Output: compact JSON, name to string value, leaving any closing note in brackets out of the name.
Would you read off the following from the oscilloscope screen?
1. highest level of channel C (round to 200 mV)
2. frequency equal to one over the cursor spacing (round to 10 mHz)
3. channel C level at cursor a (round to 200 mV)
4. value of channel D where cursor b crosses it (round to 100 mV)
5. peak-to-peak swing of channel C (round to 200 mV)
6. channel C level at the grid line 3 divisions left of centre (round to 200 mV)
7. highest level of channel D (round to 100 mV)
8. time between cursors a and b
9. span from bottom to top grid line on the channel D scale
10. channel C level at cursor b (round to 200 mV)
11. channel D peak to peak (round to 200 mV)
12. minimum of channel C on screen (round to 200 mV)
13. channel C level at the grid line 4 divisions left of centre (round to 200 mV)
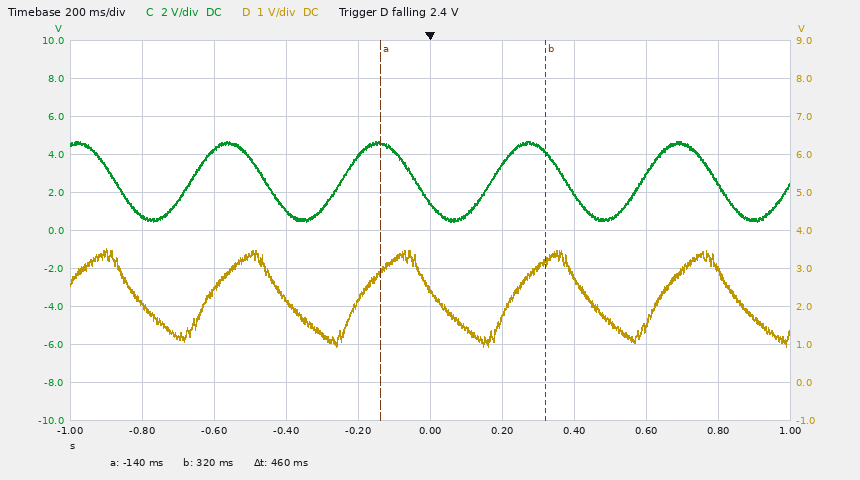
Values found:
{"highest level of channel C": "4.6 V", "frequency equal to one over the cursor spacing": "2.17 Hz", "channel C level at cursor a": "4.6 V", "value of channel D where cursor b crosses it": "3.2 V", "peak-to-peak swing of channel C": "4.2 V", "channel C level at the grid line 3 divisions left of centre": "4.2 V", "highest level of channel D": "3.5 V", "time between cursors a and b": "460 ms", "span from bottom to top grid line on the channel D scale": "10 V", "channel C level at cursor b": "4.2 V", "channel D peak to peak": "2.6 V", "minimum of channel C on screen": "400 mV", "channel C level at the grid line 4 divisions left of centre": "800 mV"}
